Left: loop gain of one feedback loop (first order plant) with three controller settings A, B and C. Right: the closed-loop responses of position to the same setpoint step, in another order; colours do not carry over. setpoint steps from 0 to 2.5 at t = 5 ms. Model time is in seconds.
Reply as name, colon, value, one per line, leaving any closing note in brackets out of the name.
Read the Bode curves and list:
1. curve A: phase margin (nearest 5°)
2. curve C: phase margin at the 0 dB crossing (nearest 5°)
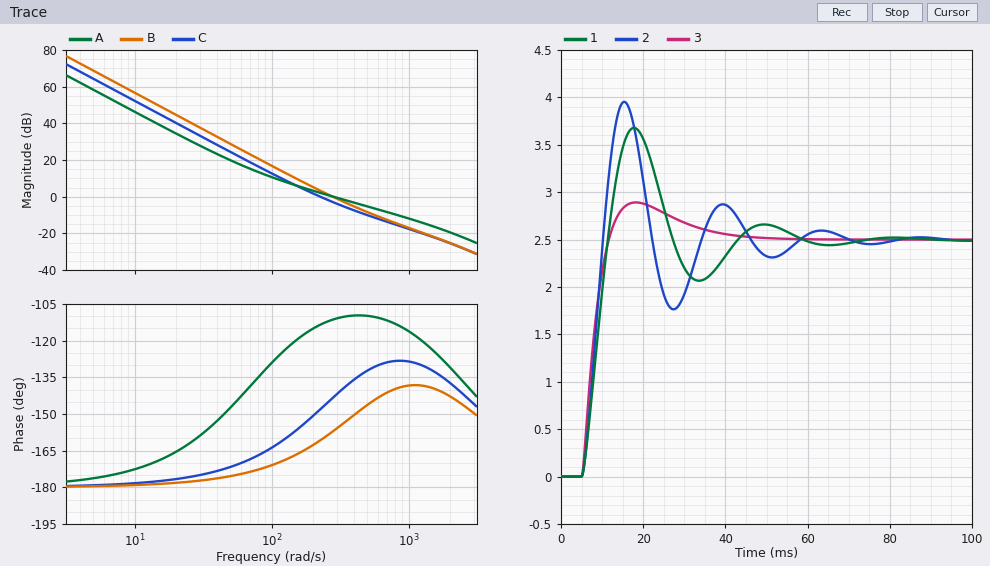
curve A: phase margin: 70°
curve C: phase margin at the 0 dB crossing: 30°
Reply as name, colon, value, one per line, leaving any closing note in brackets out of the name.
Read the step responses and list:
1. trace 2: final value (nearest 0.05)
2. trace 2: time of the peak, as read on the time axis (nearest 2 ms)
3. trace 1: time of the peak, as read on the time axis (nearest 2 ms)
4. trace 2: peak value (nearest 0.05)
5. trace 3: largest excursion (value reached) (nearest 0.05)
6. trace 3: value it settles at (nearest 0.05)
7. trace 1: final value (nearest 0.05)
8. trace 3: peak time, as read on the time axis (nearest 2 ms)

trace 2: final value: 2.50
trace 2: time of the peak, as read on the time axis: 16 ms
trace 1: time of the peak, as read on the time axis: 18 ms
trace 2: peak value: 3.95
trace 3: largest excursion (value reached): 2.90
trace 3: value it settles at: 2.50
trace 1: final value: 2.50
trace 3: peak time, as read on the time axis: 18 ms
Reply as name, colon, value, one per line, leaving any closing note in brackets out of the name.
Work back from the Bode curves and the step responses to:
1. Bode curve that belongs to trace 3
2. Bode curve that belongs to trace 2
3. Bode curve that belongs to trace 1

Bode curve that belongs to trace 3: A
Bode curve that belongs to trace 2: B
Bode curve that belongs to trace 1: C
